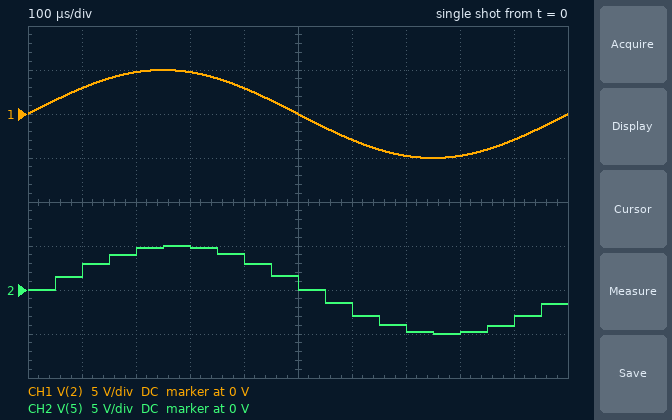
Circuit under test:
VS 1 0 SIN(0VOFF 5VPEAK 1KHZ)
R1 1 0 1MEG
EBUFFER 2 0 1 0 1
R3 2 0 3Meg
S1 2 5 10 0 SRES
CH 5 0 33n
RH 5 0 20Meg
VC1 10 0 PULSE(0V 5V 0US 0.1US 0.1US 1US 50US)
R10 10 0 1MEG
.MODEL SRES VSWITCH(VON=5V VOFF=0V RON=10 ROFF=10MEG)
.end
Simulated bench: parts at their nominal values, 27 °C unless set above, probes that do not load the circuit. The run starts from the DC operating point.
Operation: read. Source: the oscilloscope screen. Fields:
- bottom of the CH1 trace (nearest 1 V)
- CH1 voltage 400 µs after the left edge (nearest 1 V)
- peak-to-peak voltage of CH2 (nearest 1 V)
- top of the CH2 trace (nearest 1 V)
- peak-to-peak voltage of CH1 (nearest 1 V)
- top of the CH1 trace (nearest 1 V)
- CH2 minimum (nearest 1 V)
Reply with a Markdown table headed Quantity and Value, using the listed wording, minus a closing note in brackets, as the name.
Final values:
| Quantity | Value |
|---|---|
| bottom of the CH1 trace | -5 V |
| CH1 voltage 400 µs after the left edge | 3 V |
| peak-to-peak voltage of CH2 | 10 V |
| top of the CH2 trace | 5 V |
| peak-to-peak voltage of CH1 | 10 V |
| top of the CH1 trace | 5 V |
| CH2 minimum | -5 V |
